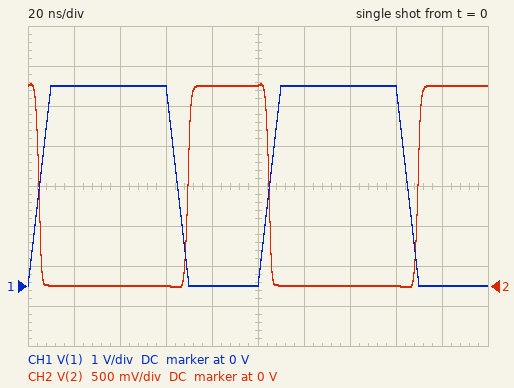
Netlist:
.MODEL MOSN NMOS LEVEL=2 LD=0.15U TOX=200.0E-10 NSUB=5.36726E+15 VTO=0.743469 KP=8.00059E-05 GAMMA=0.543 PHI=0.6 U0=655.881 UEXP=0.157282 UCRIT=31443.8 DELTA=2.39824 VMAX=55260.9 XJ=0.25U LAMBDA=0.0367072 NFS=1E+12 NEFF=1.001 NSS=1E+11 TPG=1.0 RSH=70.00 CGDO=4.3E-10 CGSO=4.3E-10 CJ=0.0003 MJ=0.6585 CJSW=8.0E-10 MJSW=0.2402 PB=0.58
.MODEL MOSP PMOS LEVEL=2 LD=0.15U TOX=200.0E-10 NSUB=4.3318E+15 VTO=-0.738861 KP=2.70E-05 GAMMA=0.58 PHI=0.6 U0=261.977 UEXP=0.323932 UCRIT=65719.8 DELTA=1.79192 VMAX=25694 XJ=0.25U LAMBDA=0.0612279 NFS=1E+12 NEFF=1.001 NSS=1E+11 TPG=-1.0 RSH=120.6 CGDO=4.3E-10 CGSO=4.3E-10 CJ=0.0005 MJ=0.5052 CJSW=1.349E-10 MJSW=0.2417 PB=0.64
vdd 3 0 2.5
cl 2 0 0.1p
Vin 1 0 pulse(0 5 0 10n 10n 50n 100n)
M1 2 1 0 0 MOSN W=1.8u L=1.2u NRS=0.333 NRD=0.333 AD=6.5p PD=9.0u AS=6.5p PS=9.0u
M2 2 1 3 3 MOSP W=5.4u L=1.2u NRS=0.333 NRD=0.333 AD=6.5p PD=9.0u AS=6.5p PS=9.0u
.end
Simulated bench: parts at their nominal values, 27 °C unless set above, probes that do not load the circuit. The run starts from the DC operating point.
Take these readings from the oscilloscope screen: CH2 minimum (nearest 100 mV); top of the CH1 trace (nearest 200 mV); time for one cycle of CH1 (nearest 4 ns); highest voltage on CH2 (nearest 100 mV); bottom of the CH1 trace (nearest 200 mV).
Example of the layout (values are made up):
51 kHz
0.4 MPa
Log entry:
0 V
5.0 V
100 ns
2.5 V
0 V
